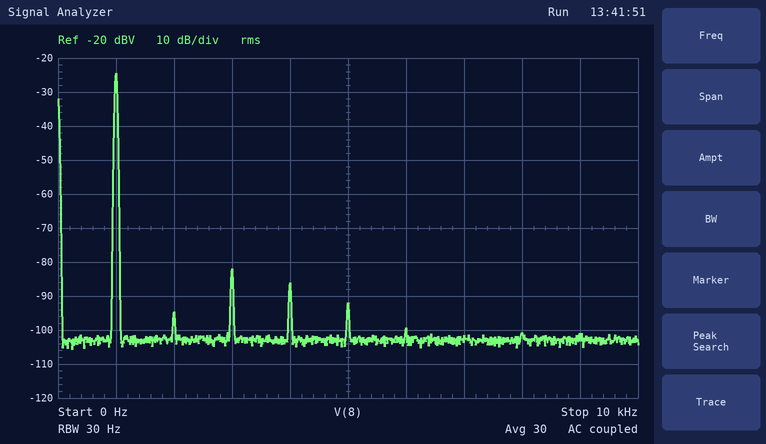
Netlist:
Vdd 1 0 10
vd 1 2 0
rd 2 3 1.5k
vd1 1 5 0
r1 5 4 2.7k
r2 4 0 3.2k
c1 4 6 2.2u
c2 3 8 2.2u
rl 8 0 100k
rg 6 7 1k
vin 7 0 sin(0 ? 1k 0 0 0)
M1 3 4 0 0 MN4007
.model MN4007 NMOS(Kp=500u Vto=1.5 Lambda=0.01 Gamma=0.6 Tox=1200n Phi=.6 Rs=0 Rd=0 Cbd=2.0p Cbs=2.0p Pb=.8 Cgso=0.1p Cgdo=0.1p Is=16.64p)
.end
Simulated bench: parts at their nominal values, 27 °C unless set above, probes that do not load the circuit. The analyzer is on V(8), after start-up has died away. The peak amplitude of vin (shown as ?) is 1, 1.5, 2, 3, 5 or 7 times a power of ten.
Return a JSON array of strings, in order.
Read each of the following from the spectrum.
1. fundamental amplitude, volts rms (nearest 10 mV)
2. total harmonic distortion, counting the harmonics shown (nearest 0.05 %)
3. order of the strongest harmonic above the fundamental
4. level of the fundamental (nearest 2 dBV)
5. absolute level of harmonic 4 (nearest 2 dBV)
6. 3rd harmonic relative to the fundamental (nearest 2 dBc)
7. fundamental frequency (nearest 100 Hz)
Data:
["60 mV", "0.15 %", "3", "-24 dBV", "-86 dBV", "-58 dBc", "1.0 kHz"]
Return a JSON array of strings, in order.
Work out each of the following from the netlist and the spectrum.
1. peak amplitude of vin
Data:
["50 mV"]
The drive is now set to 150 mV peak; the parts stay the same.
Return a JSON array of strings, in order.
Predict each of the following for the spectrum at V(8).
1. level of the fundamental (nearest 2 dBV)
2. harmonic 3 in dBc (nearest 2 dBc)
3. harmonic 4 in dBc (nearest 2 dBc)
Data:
["-16 dBV", "-40 dBc", "-54 dBc"]
